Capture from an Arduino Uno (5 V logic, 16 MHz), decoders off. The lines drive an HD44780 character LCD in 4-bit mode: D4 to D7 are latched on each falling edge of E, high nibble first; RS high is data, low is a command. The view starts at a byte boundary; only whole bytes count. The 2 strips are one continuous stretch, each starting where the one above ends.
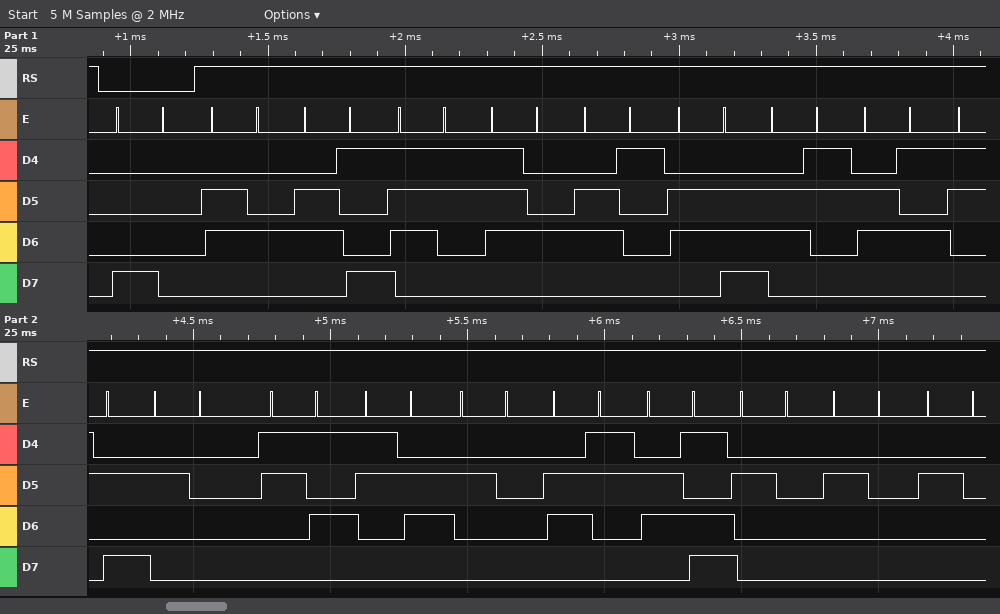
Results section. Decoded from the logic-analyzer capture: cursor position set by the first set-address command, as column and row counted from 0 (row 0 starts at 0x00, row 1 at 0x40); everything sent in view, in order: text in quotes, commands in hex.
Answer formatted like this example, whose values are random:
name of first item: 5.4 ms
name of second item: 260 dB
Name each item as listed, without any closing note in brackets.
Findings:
cursor position set by the first set-address command, as column and row counted from 0: column 0, row 0
everything sent in view, in order: text in quotes, commands in hex: 0x80 "distance: 56 cm   "
